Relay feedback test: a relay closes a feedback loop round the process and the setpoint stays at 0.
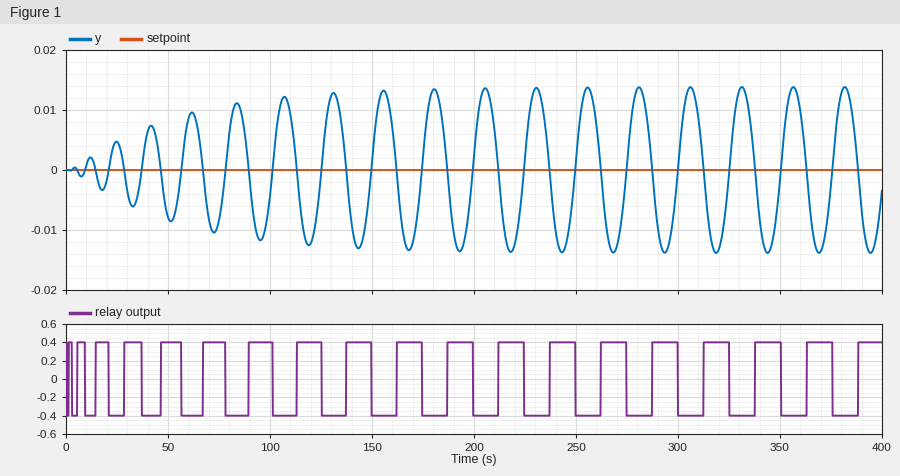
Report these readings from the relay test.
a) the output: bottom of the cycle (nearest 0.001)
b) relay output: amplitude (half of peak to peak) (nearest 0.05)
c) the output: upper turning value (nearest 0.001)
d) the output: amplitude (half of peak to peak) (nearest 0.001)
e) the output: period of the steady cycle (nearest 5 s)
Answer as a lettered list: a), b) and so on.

a) -0.014
b) 0.40
c) 0.014
d) 0.014
e) 25 s
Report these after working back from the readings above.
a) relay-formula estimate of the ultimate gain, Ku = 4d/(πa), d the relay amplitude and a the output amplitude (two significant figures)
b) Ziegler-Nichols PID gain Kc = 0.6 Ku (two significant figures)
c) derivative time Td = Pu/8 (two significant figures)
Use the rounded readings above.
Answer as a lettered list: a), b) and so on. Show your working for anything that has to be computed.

a) 4 × 0.4 / (π × 0.014) = 36
b) 0.6 × 36 = 22
c) 25 / 8 = 3.1 s
